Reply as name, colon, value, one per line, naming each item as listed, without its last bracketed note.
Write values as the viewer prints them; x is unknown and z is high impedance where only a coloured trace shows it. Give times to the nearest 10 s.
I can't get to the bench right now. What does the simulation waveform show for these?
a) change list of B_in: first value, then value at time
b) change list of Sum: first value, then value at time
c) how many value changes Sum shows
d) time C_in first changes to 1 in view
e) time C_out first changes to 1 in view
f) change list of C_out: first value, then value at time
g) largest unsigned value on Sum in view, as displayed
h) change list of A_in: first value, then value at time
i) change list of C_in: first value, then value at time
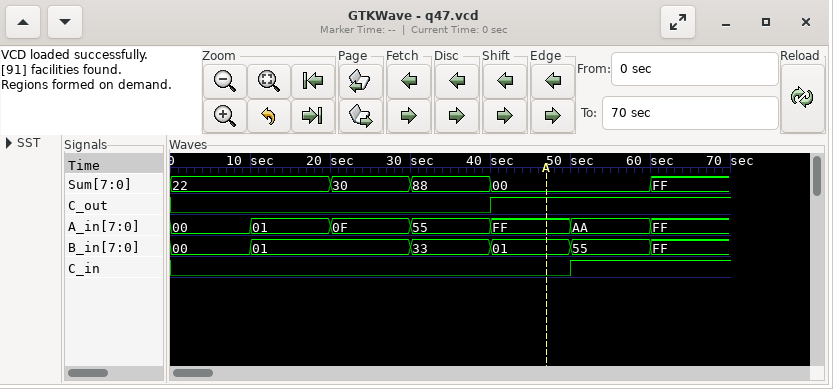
change list of B_in: first value, then value at time: 00, 01 at 10 s, 33 at 30 s, 01 at 40 s, 55 at 50 s, FF at 60 s
change list of Sum: first value, then value at time: 22, 30 at 20 s, 88 at 30 s, 00 at 40 s, FF at 60 s
how many value changes Sum shows: 4
time C_in first changes to 1 in view: 50 s
time C_out first changes to 1 in view: 40 s
change list of C_out: first value, then value at time: 0, 1 at 40 s
largest unsigned value on Sum in view, as displayed: FF
change list of A_in: first value, then value at time: 00, 01 at 10 s, 0F at 20 s, 55 at 30 s, FF at 40 s, AA at 50 s, FF at 60 s
change list of C_in: first value, then value at time: 0, 1 at 50 s
